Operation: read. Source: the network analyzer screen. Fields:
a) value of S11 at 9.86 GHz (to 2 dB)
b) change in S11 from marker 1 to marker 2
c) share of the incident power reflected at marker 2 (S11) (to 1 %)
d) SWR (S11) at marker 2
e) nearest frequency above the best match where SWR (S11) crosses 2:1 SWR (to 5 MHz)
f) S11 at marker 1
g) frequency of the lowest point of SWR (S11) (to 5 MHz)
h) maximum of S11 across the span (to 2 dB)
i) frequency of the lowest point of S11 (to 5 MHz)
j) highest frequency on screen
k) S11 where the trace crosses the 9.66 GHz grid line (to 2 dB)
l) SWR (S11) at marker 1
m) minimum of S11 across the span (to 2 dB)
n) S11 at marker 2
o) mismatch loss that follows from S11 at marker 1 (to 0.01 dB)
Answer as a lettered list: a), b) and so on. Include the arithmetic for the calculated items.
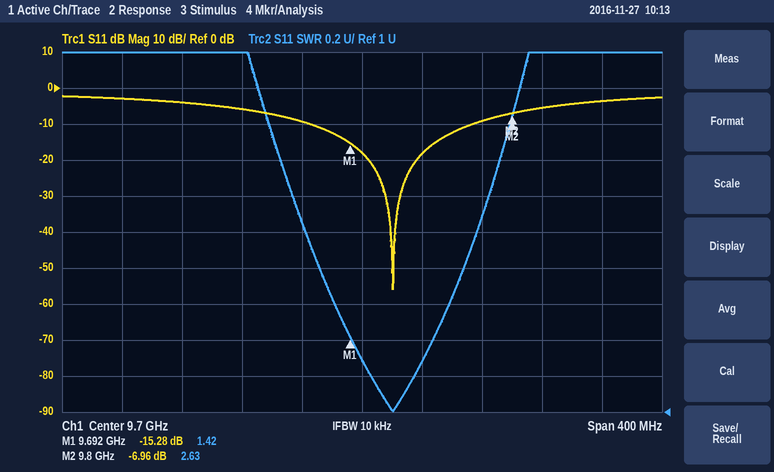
a) -4 dB
b) -6.96 − (-15.28) = 8.32 dB
c) 10^(-6.96/10) ≈ 20 %
d) 2.63
e) 9.775 GHz
f) -15.28 dB
g) 9.720 GHz
h) -2 dB
i) 9.720 GHz
j) 9.9 GHz
k) -10 dB
l) 1.42
m) -56 dB
n) -6.96 dB
o) −10 log10(1 − 10^(-15.28/10)) ≈ 0.13 dB
